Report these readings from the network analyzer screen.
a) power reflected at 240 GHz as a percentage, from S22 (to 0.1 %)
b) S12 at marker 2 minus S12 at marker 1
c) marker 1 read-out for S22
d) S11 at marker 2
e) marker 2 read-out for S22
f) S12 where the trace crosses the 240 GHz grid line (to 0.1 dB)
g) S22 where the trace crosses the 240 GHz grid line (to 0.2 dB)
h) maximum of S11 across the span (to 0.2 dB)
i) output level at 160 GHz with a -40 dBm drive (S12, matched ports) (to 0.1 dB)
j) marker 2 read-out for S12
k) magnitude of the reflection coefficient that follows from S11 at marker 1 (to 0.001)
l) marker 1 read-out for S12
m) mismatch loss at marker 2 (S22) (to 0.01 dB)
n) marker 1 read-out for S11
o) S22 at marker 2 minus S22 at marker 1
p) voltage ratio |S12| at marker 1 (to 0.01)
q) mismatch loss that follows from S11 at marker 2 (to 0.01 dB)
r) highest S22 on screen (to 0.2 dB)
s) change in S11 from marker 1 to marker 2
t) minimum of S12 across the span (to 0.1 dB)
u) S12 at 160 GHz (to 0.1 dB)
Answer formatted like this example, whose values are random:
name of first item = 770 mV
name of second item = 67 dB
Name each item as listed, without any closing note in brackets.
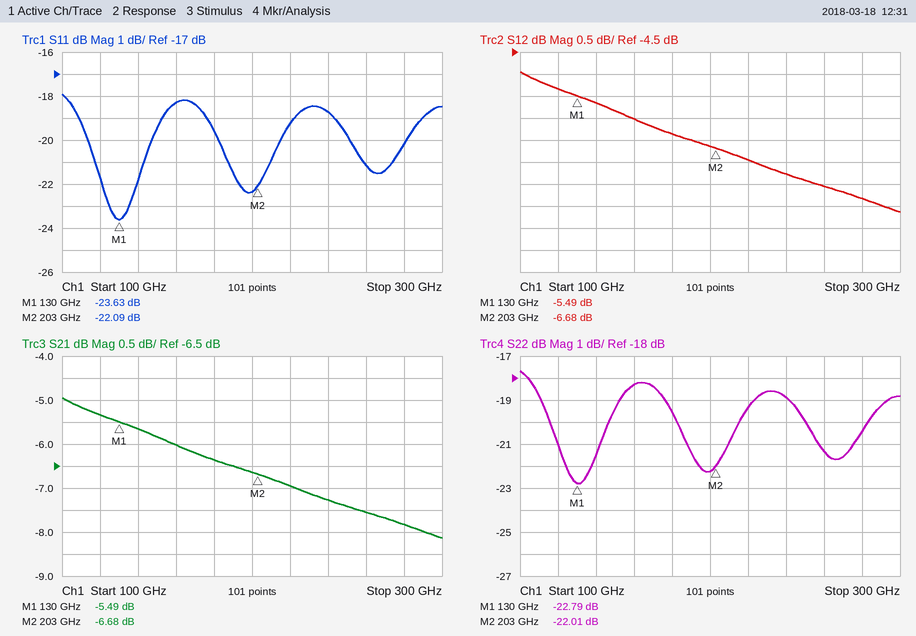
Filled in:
power reflected at 240 GHz as a percentage, from S22 = 1.3 %
S12 at marker 2 minus S12 at marker 1 = -1.19 dB
marker 1 read-out for S22 = -22.79 dB
S11 at marker 2 = -22.09 dB
marker 2 read-out for S22 = -22.01 dB
S12 where the trace crosses the 240 GHz grid line = -7.3 dB
S22 where the trace crosses the 240 GHz grid line = -18.8 dB
maximum of S11 across the span = -18.0 dB
output level at 160 GHz with a -40 dBm drive (S12, matched ports) = -46.0 dBm
marker 2 read-out for S12 = -6.68 dB
magnitude of the reflection coefficient that follows from S11 at marker 1 = 0.066
marker 1 read-out for S12 = -5.49 dB
mismatch loss at marker 2 (S22) = 0.03 dB
marker 1 read-out for S11 = -23.63 dB
S22 at marker 2 minus S22 at marker 1 = 0.78 dB
voltage ratio |S12| at marker 1 = 0.53
mismatch loss that follows from S11 at marker 2 = 0.03 dB
highest S22 on screen = -17.6 dB
change in S11 from marker 1 to marker 2 = 1.54 dB
minimum of S12 across the span = -8.1 dB
S12 at 160 GHz = -6.0 dB
